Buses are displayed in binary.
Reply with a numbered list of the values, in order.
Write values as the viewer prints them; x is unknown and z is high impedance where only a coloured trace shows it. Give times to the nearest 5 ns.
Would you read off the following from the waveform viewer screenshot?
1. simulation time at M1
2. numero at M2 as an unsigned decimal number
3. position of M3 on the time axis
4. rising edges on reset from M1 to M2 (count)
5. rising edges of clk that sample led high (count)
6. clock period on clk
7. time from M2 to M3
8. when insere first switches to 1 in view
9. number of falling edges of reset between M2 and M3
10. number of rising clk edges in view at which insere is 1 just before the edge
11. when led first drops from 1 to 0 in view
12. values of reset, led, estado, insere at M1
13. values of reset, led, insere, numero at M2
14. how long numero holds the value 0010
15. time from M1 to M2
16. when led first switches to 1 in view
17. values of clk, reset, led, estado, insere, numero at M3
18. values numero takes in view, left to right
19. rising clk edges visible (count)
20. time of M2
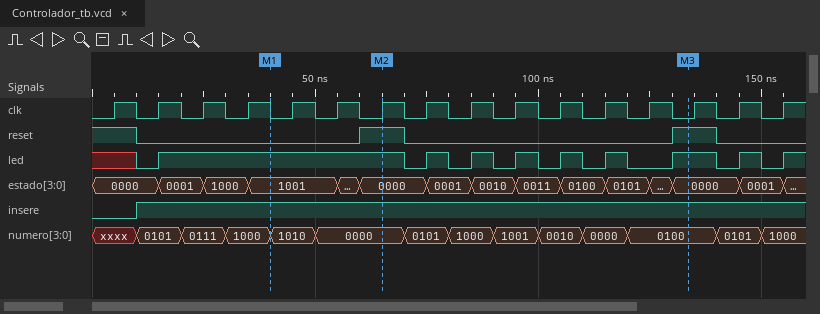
1. 40 ns
2. 0
3. 135 ns
4. 1
5. 6
6. 10 ns
7. 70 ns
8. 10 ns
9. 1
10. 15
11. 70 ns
12. reset=0, led=1, estado=1001, insere=1
13. reset=1, led=1, insere=1, numero=0000
14. 10 ns
15. 25 ns
16. 15 ns
17. clk=0, reset=1, led=1, estado=0000, insere=1, numero=0100
18. xxxx, 0101, 0111, 1000, 1010, 0000, 0101, 1000, 1001, 0010, 0000, 0100, 0101, 1000
19. 16
20. 65 ns
